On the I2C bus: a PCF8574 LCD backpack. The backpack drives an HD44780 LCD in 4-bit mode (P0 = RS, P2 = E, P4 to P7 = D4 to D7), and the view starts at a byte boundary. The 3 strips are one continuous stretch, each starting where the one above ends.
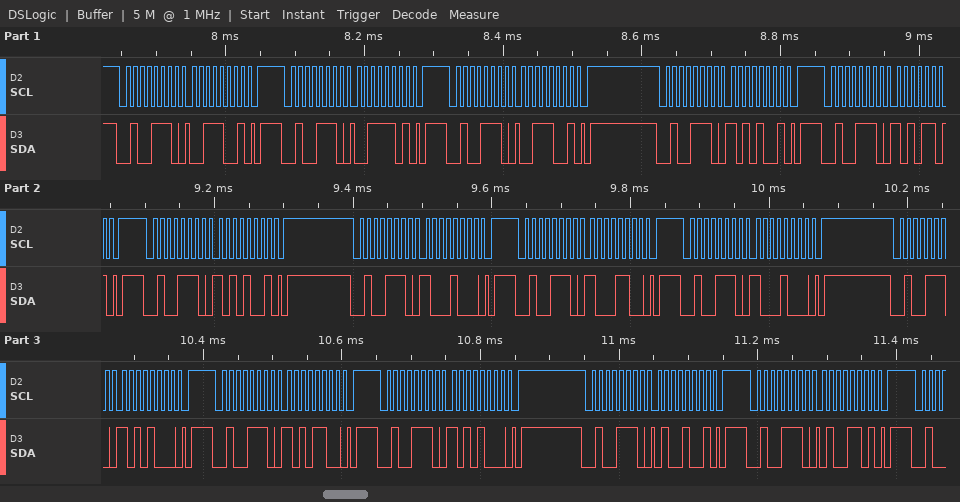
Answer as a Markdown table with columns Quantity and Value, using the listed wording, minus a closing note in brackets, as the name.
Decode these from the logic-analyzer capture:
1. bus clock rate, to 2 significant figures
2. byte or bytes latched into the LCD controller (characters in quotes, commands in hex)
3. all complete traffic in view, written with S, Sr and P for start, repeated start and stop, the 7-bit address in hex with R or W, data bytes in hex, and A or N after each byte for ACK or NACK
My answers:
| Quantity | Value |
|---|---|
| bus clock rate, to 2 significant figures | 100 kHz |
| byte or bytes latched into the LCD controller | ':' 0x8A |
| all complete traffic in view, written with S, Sr and P for start, repeated start and stop, the 7-bit address in hex with R or W, data bytes in hex, and A or N after each byte for ACK or NACK | S 27W A 39 A P S 27W A 3D A P S 27W A 39 A P S 27W A A9 A P S 27W A AD A P S 27W A A9 A P S 27W A 88 A P S 27W A 8C A P S 27W A 88 A P S 27W A A8 A P S 27W A AC A P S 27W A A8 A P S 27W A 49 A P S 27W A 4D A P |
